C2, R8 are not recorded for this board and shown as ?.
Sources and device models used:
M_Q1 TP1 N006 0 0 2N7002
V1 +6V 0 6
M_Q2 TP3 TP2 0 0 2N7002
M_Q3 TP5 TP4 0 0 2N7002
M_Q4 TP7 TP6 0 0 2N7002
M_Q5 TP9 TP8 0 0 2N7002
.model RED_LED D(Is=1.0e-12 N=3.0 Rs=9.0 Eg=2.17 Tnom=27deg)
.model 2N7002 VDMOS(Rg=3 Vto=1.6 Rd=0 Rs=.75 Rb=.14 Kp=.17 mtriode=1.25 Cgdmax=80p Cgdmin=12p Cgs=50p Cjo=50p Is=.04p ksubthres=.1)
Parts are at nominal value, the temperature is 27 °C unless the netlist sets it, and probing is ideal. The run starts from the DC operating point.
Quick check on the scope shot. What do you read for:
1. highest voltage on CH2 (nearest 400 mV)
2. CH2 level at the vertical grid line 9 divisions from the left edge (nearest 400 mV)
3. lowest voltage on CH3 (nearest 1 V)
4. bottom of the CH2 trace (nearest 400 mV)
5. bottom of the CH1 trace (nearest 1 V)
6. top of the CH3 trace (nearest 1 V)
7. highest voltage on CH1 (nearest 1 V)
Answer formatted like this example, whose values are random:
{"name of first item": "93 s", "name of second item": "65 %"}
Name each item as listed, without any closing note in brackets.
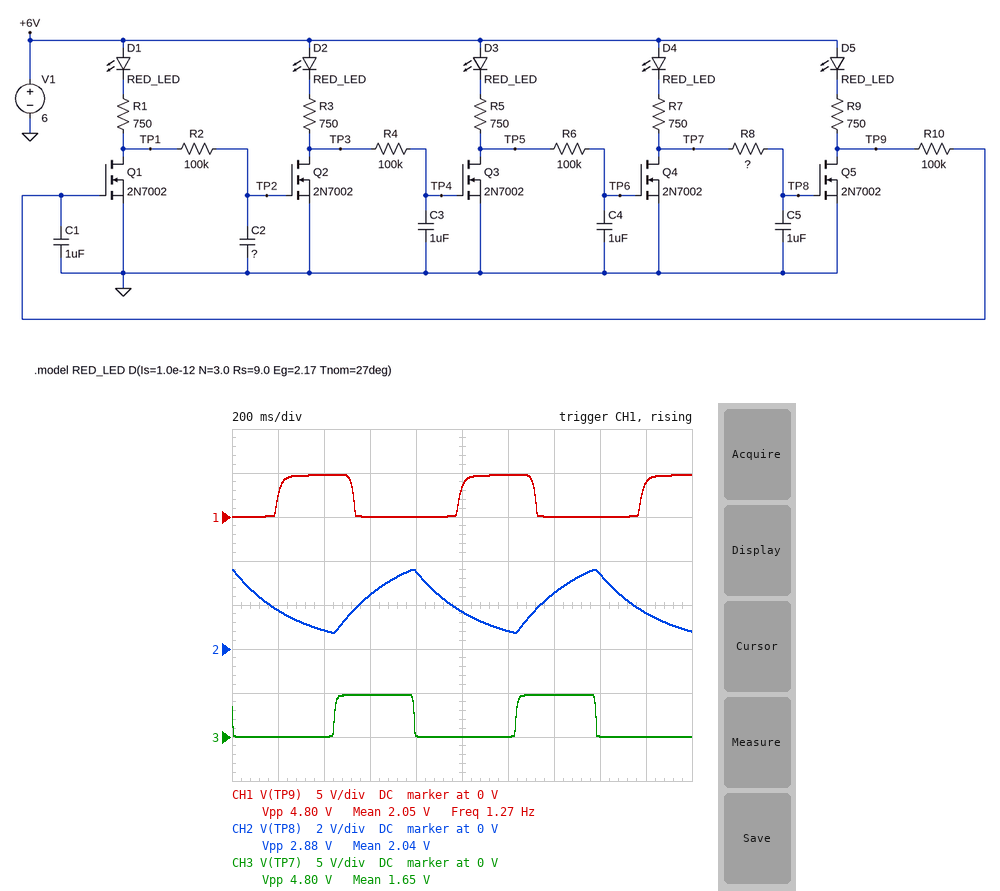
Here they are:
{"highest voltage on CH2": "3.6 V", "CH2 level at the vertical grid line 9 divisions from the left edge": "1.6 V", "lowest voltage on CH3": "0 V", "bottom of the CH2 trace": "800 mV", "bottom of the CH1 trace": "0 V", "top of the CH3 trace": "5 V", "highest voltage on CH1": "5 V"}
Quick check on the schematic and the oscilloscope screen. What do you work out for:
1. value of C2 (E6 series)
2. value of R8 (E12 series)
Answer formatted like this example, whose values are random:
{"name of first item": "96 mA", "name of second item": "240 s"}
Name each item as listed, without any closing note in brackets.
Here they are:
{"value of C2": "470 nF", "value of R8": "270 kΩ"}
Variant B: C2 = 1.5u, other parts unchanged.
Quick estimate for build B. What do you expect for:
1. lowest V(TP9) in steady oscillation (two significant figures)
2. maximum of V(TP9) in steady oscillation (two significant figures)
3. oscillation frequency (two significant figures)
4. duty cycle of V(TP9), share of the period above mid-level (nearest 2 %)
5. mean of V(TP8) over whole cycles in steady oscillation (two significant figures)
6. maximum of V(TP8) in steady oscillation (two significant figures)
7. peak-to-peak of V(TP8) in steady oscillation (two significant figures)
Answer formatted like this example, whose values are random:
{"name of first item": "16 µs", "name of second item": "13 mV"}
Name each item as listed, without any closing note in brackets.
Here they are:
{"lowest V(TP9) in steady oscillation": "16 mV", "maximum of V(TP9) in steady oscillation": "4.9 V", "oscillation frequency": "1.0 Hz", "duty cycle of V(TP9), share of the period above mid-level": "46 %", "mean of V(TP8) over whole cycles in steady oscillation": "2.0 V", "maximum of V(TP8) in steady oscillation": "3.8 V", "peak-to-peak of V(TP8) in steady oscillation": "3.3 V"}
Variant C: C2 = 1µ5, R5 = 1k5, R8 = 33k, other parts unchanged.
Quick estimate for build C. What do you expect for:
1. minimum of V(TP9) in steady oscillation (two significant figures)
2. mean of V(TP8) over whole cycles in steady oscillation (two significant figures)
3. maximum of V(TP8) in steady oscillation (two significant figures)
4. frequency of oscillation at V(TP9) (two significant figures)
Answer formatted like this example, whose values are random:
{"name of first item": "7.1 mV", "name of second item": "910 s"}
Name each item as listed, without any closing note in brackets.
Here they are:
{"minimum of V(TP9) in steady oscillation": "12 mV", "mean of V(TP8) over whole cycles in steady oscillation": "2.3 V", "maximum of V(TP8) in steady oscillation": "4.9 V", "frequency of oscillation at V(TP9)": "1.5 Hz"}
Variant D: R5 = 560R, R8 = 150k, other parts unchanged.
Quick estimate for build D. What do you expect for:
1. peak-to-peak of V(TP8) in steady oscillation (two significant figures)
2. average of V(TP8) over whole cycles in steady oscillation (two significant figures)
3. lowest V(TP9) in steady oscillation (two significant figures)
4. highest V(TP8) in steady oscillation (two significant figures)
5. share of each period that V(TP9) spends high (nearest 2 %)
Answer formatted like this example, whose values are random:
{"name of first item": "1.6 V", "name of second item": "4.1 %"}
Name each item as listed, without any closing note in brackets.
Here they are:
{"peak-to-peak of V(TP8) in steady oscillation": "3.8 V", "average of V(TP8) over whole cycles in steady oscillation": "2.2 V", "lowest V(TP9) in steady oscillation": "14 mV", "highest V(TP8) in steady oscillation": "4.2 V", "share of each period that V(TP9) spends high": "44 %"}
